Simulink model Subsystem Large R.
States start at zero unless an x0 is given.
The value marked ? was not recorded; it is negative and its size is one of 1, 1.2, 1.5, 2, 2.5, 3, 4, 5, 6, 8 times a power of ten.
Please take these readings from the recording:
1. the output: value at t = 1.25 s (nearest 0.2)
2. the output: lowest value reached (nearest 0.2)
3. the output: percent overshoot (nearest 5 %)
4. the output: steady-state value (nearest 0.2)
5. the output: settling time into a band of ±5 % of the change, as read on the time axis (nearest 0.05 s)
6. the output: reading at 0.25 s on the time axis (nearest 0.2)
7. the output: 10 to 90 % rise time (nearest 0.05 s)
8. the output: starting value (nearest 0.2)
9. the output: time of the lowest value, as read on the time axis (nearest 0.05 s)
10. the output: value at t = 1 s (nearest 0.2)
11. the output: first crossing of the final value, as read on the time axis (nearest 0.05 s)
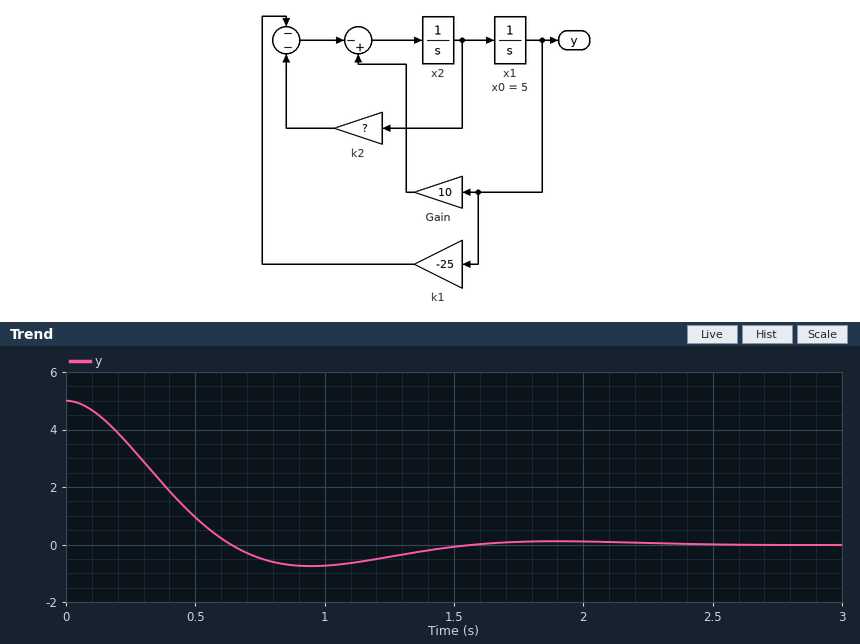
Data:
-0.4
-0.8
15 %
0.0
1.35 s
3.4
0.45 s
5.0
0.95 s
-0.8
0.65 s
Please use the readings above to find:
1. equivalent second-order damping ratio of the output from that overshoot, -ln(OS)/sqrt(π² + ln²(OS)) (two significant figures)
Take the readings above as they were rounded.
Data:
0.52
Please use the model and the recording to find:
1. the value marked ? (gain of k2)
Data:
-4
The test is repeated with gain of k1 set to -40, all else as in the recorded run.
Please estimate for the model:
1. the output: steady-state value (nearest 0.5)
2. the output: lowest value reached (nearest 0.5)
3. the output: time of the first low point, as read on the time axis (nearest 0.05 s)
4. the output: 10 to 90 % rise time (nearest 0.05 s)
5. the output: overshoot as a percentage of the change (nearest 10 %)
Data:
0.0
-1.5
0.60 s
0.25 s
30 %
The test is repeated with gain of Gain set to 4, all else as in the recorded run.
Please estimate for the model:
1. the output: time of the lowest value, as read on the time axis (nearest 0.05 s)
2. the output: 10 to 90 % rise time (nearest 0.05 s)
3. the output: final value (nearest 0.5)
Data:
0.75 s
0.35 s
0.0
